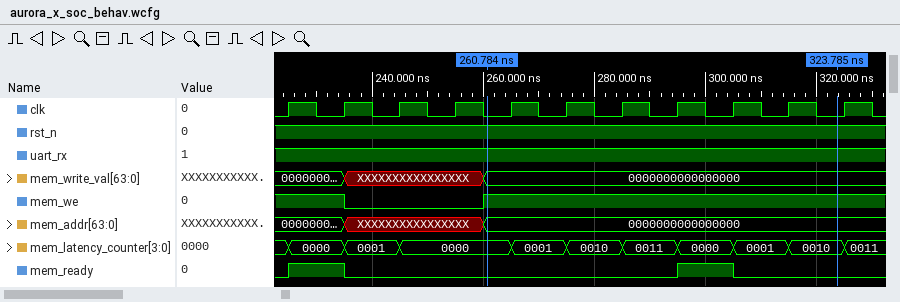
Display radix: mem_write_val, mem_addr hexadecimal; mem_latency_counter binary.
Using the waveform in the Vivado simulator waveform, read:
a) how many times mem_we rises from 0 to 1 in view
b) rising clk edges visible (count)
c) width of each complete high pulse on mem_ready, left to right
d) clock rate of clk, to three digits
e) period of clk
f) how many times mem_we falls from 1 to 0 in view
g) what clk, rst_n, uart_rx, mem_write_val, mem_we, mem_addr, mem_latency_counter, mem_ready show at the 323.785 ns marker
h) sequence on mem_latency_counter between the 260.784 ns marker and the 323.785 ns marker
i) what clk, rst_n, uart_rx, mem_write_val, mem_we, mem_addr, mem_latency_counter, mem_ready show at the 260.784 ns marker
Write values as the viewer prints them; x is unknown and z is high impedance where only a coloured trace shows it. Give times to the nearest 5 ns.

1
11
10 ns, 10 ns
100 MHz
10 ns
1
clk=0, rst_n=1, uart_rx=1, mem_write_val=0000000000000000, mem_we=1, mem_addr=0000000000000000, mem_latency_counter=0010, mem_ready=0
0000, 0001, 0010, 0011, 0000, 0001, 0010
clk=0, rst_n=1, uart_rx=1, mem_write_val=0000000000000000, mem_we=1, mem_addr=0000000000000000, mem_latency_counter=0000, mem_ready=0
